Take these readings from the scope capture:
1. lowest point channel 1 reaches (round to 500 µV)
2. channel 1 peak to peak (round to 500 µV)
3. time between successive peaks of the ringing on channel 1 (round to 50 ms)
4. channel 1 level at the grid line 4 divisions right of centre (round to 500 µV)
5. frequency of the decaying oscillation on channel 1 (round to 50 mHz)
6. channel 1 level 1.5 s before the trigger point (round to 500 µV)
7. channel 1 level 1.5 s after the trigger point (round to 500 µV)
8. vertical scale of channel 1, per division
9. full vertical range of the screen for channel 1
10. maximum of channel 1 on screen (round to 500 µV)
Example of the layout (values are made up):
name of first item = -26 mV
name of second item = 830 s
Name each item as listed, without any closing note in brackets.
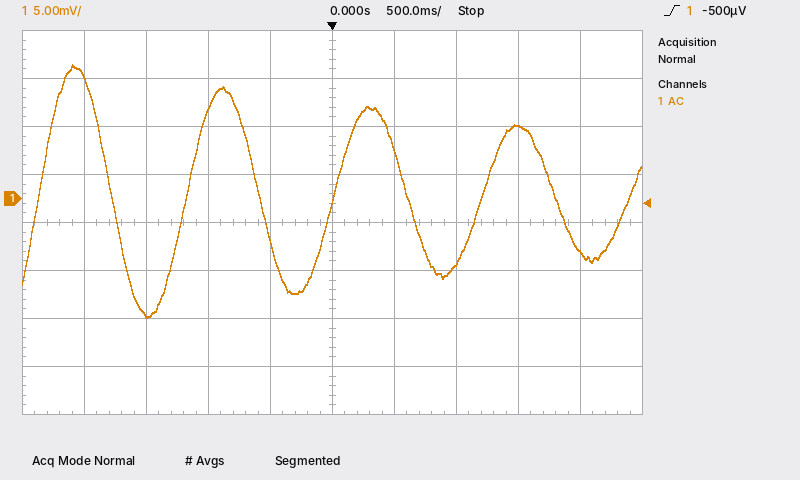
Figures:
lowest point channel 1 reaches = -12.5 mV
channel 1 peak to peak = 26.5 mV
time between successive peaks of the ringing on channel 1 = 1.20 s
channel 1 level at the grid line 4 divisions right of centre = -5.5 mV
frequency of the decaying oscillation on channel 1 = 850 mHz
channel 1 level 1.5 s before the trigger point = -12.0 mV
channel 1 level 1.5 s after the trigger point = 7.5 mV
vertical scale of channel 1, per division = 5 mV
full vertical range of the screen for channel 1 = 40 mV
maximum of channel 1 on screen = 14.0 mV
